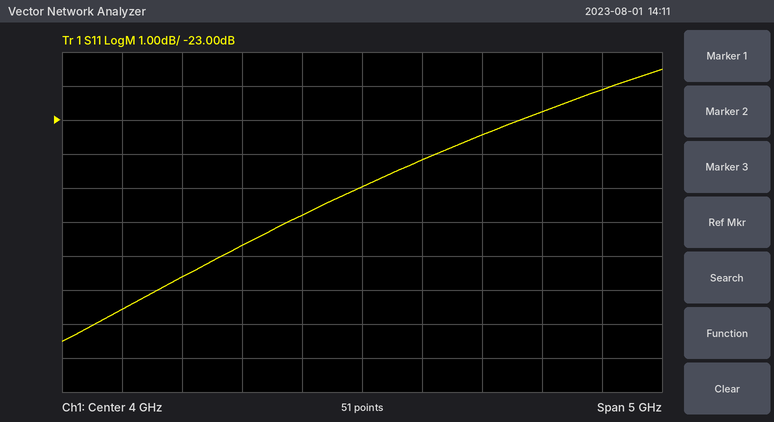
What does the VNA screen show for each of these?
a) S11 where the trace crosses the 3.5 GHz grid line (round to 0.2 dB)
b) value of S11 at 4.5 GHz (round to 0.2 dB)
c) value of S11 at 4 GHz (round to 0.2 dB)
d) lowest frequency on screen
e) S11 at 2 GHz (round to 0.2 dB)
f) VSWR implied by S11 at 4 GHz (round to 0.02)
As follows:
-25.8 dB
-24.2 dB
-25.0 dB
1.5 GHz
-28.6 dB
1.12
